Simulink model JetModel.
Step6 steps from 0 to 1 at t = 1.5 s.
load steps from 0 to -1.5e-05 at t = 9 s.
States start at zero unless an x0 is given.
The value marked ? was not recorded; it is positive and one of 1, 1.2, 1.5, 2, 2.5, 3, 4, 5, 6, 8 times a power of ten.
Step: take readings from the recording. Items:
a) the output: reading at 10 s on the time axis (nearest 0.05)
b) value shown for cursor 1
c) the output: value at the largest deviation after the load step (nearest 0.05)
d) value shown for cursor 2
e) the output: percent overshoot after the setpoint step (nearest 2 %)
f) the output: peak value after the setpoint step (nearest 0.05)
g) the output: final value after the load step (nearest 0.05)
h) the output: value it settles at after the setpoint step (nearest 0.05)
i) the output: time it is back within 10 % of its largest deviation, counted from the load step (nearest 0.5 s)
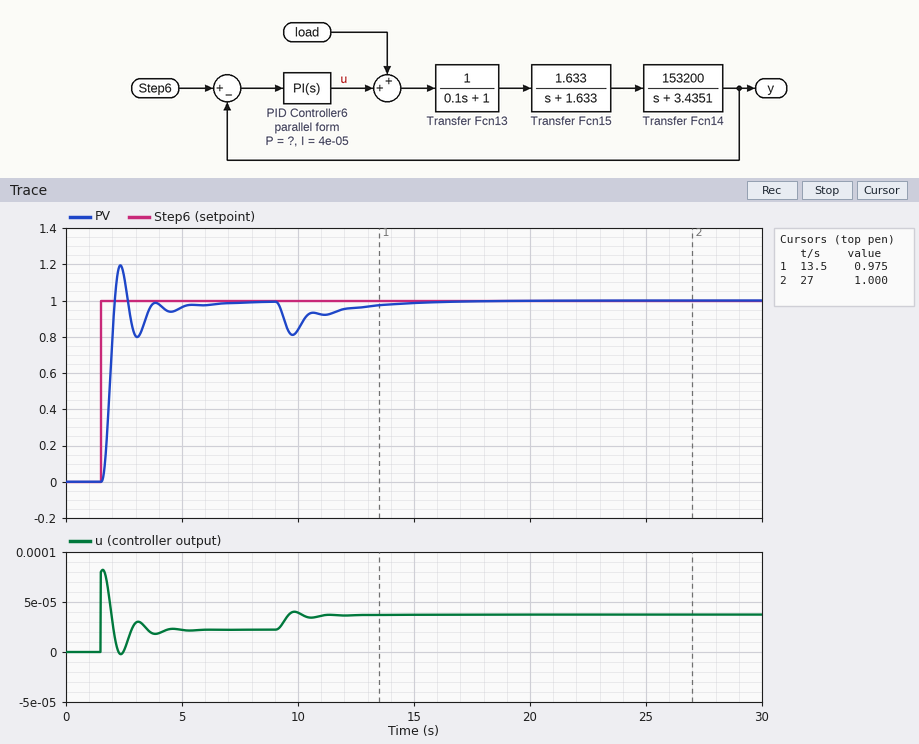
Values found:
0.85
0.975
0.80
1.000
20 %
1.20
1.00
1.00
5.5 s
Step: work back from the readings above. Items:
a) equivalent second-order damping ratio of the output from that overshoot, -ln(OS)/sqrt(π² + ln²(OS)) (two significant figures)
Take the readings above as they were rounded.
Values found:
0.46
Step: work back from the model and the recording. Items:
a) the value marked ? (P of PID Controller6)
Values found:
8e-05
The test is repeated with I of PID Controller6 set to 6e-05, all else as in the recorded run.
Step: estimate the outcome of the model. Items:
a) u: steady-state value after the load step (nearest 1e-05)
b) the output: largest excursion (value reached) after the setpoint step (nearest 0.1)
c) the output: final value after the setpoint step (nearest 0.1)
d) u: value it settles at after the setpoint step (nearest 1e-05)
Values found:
0.00004
1.3
1.0
0.00002
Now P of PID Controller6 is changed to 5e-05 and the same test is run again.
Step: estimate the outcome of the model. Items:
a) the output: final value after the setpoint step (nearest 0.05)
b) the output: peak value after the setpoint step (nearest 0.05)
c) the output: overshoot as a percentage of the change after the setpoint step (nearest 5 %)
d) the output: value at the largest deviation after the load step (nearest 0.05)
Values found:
1.00
1.10
10 %
0.75
